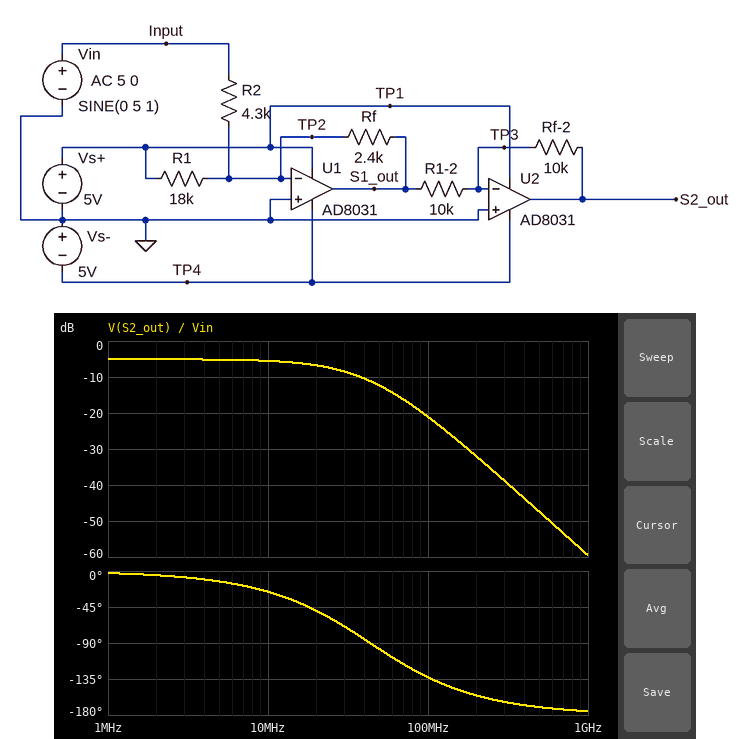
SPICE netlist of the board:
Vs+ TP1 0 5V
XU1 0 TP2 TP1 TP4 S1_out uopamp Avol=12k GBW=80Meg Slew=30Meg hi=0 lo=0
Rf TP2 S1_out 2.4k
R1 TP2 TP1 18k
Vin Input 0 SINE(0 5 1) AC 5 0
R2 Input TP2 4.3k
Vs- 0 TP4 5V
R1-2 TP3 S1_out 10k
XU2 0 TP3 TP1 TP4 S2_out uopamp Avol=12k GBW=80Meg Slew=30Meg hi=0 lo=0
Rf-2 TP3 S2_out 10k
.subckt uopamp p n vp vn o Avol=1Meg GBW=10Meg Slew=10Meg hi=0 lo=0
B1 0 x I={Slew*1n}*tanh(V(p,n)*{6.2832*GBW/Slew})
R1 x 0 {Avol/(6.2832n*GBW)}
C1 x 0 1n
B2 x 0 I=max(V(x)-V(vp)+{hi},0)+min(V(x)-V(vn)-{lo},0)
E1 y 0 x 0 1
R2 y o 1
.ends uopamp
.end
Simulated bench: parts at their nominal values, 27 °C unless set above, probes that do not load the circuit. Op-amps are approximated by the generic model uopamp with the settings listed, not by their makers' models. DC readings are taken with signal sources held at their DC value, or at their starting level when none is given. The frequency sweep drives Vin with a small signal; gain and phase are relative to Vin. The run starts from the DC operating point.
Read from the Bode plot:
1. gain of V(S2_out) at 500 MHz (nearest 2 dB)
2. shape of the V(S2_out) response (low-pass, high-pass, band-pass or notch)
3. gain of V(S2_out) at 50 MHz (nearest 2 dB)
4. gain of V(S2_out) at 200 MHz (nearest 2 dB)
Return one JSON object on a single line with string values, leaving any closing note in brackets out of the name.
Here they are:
{"gain of V(S2_out) at 500 MHz": "-48 dB", "shape of the V(S2_out) response": "low-pass", "gain of V(S2_out) at 50 MHz": "-12 dB", "gain of V(S2_out) at 200 MHz": "-32 dB"}
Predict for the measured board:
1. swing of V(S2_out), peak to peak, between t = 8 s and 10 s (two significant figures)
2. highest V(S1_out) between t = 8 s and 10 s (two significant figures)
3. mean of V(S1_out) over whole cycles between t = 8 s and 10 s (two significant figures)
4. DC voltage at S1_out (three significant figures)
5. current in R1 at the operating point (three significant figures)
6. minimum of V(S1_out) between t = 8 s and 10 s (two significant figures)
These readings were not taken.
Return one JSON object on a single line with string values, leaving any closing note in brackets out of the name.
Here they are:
{"swing of V(S2_out), peak to peak, between t = 8 s and 10 s": "5.6 V", "highest V(S1_out) between t = 8 s and 10 s": "2.1 V", "mean of V(S1_out) over whole cycles between t = 8 s and 10 s": "-670 mV", "DC voltage at S1_out": "-667 mV", "current in R1 at the operating point": "278 µA", "minimum of V(S1_out) between t = 8 s and 10 s": "-3.5 V"}
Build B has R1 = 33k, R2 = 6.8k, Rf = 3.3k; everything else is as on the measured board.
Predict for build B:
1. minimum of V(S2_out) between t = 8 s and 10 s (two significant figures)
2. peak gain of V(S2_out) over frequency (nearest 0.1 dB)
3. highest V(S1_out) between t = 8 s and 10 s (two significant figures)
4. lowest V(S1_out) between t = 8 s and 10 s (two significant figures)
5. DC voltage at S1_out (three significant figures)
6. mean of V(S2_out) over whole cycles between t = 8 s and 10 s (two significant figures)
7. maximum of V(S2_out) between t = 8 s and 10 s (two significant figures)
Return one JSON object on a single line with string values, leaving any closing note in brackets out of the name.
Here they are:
{"minimum of V(S2_out) between t = 8 s and 10 s": "-1.9 V", "peak gain of V(S2_out) over frequency": "-6.3 dB", "highest V(S1_out) between t = 8 s and 10 s": "1.9 V", "lowest V(S1_out) between t = 8 s and 10 s": "-2.9 V", "DC voltage at S1_out": "-500 mV", "mean of V(S2_out) over whole cycles between t = 8 s and 10 s": "500 mV", "maximum of V(S2_out) between t = 8 s and 10 s": "2.9 V"}
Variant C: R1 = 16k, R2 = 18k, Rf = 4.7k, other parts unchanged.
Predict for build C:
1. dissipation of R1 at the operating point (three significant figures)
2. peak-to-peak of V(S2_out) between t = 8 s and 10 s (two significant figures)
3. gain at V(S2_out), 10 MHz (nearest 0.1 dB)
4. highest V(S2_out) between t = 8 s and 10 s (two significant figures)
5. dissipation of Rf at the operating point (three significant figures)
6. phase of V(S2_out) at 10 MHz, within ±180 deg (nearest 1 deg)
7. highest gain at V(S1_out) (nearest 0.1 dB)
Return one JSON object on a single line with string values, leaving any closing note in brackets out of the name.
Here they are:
{"dissipation of R1 at the operating point": "1.56 mW", "peak-to-peak of V(S2_out) between t = 8 s and 10 s": "2.6 V", "gain at V(S2_out), 10 MHz": "-12.1 dB", "highest V(S2_out) between t = 8 s and 10 s": "2.8 V", "dissipation of Rf at the operating point": "459 µW", "phase of V(S2_out) at 10 MHz, within ±180 deg": "-25 deg", "highest gain at V(S1_out)": "-11.7 dB"}
